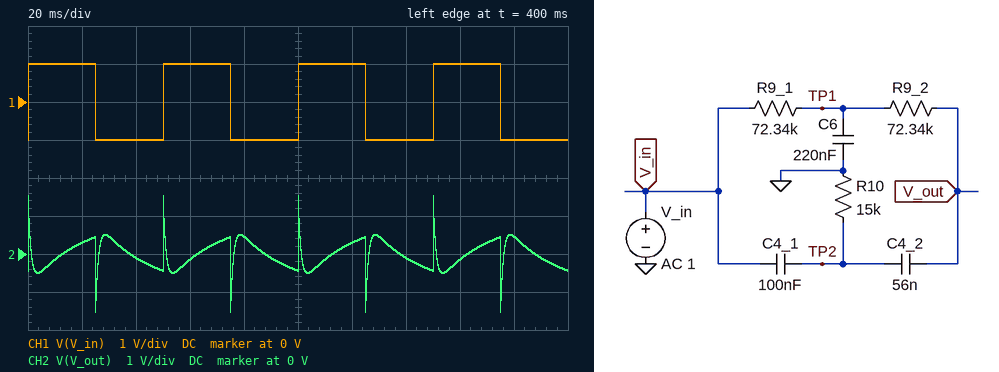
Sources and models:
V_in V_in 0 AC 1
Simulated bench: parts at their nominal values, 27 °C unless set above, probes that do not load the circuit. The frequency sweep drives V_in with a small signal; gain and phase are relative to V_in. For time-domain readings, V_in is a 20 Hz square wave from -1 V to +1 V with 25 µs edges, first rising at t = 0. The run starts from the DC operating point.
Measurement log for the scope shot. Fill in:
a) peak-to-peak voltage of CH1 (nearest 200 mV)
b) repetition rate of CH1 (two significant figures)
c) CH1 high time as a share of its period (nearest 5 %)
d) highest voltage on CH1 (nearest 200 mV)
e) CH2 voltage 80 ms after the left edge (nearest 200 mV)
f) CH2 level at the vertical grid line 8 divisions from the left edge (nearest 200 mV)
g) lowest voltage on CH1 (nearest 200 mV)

2.0 V
20 Hz
50 %
1.0 V
400 mV
-200 mV
-1.0 V
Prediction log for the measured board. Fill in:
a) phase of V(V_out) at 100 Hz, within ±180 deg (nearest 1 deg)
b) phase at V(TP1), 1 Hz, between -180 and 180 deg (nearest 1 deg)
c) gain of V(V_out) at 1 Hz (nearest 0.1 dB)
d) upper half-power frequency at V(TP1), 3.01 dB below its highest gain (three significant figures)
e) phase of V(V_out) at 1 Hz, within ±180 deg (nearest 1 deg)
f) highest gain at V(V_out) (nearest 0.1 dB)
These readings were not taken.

71 deg
-7 deg
-0.1 dB
7.50 Hz
-9 deg
0 dB
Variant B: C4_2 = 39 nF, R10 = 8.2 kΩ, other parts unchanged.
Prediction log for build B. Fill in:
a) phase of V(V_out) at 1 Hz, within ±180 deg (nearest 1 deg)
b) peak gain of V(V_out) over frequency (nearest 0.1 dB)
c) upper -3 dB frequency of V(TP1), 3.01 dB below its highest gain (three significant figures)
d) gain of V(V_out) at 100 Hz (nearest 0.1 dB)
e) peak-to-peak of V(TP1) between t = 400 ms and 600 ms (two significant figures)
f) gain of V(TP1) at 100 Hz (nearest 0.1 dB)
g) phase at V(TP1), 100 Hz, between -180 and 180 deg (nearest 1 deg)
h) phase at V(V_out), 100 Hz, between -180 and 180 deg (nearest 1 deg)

-8 deg
0 dB
8.22 Hz
-9.8 dB
1.2 V
-20.0 dB
-60 deg
96 deg
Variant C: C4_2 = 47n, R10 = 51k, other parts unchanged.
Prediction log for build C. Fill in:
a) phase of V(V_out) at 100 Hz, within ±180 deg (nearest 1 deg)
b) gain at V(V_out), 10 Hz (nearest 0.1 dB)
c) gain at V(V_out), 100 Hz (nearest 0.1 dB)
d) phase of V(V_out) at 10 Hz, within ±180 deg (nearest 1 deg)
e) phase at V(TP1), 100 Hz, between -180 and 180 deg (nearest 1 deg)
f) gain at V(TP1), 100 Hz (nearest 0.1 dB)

47 deg
-5.7 dB
-3.3 dB
-59 deg
-60 deg
-16.4 dB
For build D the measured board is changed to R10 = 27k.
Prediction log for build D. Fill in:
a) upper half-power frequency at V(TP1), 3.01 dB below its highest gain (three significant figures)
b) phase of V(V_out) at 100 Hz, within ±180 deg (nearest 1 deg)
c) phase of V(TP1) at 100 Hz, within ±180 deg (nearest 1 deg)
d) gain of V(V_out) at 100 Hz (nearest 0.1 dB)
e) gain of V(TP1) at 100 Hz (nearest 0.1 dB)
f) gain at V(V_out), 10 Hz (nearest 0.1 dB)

7.35 Hz
56 deg
-57 deg
-3.9 dB
-16.9 dB
-5.5 dB
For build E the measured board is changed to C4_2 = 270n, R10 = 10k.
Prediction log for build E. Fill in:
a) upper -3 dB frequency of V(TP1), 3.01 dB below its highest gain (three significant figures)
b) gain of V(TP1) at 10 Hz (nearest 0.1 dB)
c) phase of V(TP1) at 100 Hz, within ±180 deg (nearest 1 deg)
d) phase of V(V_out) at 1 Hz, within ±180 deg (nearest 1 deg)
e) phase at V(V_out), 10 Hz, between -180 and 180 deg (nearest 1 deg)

3.78 Hz
-6.7 dB
-59 deg
-19 deg
-89 deg
